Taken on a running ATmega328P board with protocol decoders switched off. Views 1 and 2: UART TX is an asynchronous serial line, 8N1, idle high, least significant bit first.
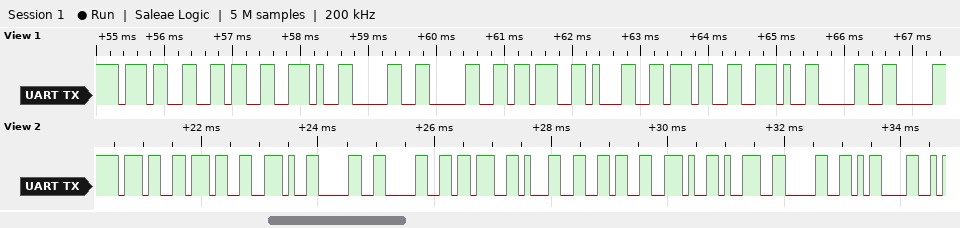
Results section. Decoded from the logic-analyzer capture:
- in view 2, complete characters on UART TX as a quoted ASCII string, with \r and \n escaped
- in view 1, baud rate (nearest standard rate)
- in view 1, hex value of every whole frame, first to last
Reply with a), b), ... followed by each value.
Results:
a) "77.00;16.90\r"
b) 9600 baud
c) 0x37 0x36 0x2E 0x30 0x30 0x3B 0x31 0x37 0x2E 0x30
